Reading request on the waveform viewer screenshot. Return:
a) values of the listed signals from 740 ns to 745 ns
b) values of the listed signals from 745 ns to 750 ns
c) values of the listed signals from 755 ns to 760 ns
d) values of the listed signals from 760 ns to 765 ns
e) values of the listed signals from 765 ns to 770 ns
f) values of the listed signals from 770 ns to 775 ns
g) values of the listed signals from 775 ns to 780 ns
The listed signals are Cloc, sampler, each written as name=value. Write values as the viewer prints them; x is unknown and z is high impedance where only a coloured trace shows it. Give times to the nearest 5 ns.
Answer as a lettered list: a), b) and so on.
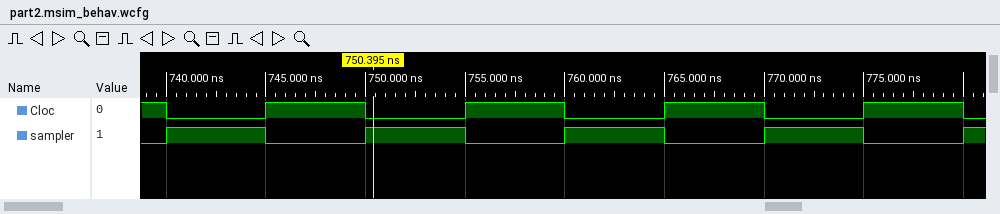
a) Cloc=0, sampler=1
b) Cloc=1, sampler=0
c) Cloc=1, sampler=0
d) Cloc=0, sampler=1
e) Cloc=1, sampler=0
f) Cloc=0, sampler=1
g) Cloc=1, sampler=0
